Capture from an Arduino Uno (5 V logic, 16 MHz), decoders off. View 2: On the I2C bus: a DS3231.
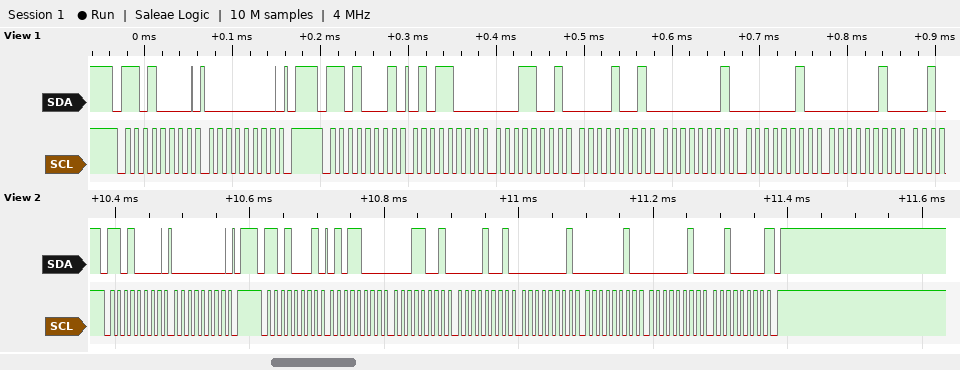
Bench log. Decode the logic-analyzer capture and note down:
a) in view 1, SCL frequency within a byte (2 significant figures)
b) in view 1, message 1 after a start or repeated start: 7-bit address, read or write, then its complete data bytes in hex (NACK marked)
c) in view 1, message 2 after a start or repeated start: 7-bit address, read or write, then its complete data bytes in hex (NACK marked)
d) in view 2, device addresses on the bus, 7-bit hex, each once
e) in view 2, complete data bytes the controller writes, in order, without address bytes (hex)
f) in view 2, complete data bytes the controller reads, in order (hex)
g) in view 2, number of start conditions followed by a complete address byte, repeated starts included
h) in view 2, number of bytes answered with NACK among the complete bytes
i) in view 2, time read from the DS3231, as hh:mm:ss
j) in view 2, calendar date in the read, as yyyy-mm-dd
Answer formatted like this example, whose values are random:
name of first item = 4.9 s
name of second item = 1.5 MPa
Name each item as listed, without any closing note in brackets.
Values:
in view 1, SCL frequency within a byte = 100 kHz
in view 1, message 1 after a start or repeated start: 7-bit address, read or write, then its complete data bytes in hex = 0x68 write: 00
in view 1, message 2 after a start or repeated start: 7-bit address, read or write, then its complete data bytes in hex = 0x68 read: 58 19 09 01 02 02
in view 2, device addresses on the bus, 7-bit hex, each once = 0x68
in view 2, complete data bytes the controller writes, in order, without address bytes = 00
in view 2, complete data bytes the controller reads, in order = 58 19 09 01 02 02 20
in view 2, number of start conditions followed by a complete address byte, repeated starts included = 2
in view 2, number of bytes answered with NACK among the complete bytes = 1
in view 2, time read from the DS3231, as hh:mm:ss = 09:19:58
in view 2, calendar date in the read, as yyyy-mm-dd = 2020-02-02
